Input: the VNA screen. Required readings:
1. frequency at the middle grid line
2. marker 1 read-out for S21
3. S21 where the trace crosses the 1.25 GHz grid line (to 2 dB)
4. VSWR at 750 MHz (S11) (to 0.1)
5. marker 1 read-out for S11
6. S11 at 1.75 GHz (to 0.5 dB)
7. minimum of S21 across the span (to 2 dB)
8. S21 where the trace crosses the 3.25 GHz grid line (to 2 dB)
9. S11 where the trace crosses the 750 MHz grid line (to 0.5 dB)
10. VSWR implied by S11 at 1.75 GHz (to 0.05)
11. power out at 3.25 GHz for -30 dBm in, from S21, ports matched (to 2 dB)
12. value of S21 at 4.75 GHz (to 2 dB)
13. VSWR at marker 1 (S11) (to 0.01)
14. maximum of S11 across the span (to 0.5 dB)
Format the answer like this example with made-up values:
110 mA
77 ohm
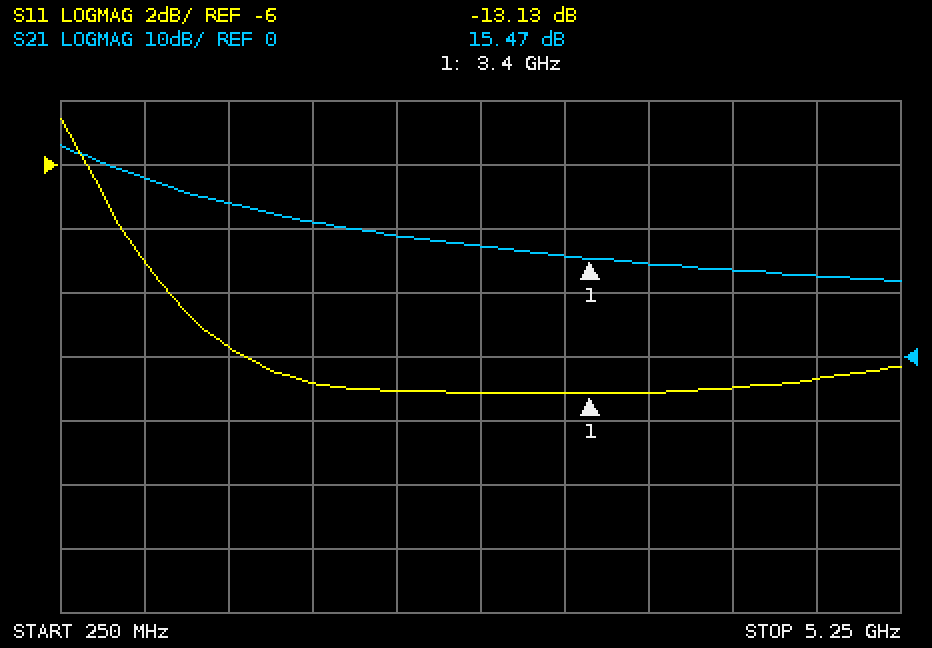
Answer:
2.75 GHz
15.47 dB
24 dB
2.1
-13.13 dB
-13.0 dB
12 dB
16 dB
-9.0 dB
1.60
-14 dBm
12 dB
1.57
-4.5 dB
